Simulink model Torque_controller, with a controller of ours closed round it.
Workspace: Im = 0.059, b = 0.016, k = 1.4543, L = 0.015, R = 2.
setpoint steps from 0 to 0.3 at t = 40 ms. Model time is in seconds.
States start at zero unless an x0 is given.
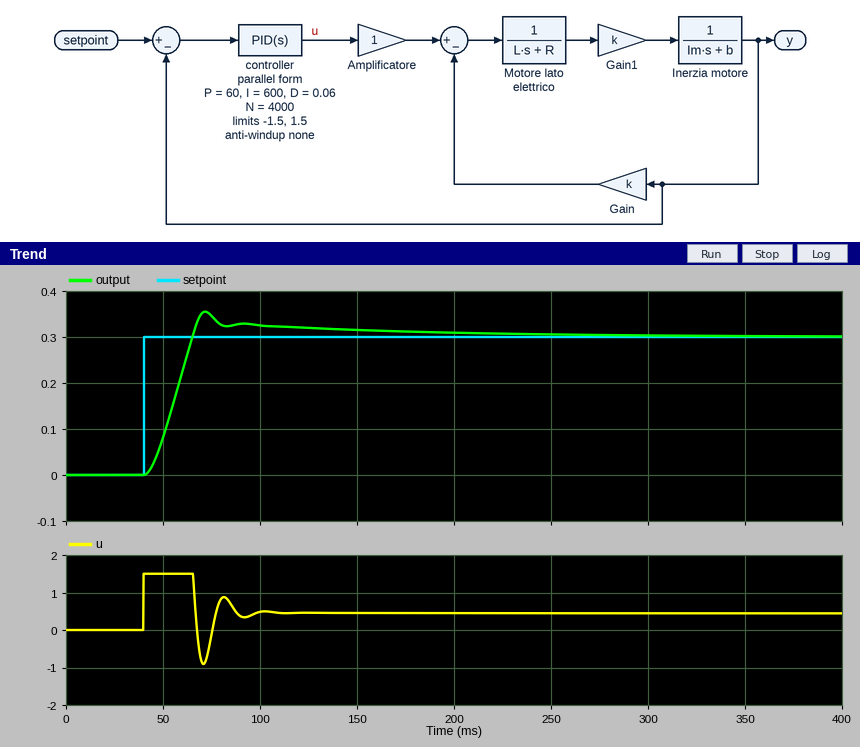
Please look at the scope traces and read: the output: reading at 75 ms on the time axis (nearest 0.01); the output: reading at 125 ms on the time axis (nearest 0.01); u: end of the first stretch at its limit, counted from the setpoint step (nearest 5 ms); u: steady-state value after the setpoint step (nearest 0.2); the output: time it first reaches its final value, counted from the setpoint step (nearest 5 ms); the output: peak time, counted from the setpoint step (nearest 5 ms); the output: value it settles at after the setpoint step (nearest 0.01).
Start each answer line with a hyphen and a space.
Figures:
- 0.35
- 0.32
- 25 ms
- 0.4
- 25 ms
- 30 ms
- 0.30
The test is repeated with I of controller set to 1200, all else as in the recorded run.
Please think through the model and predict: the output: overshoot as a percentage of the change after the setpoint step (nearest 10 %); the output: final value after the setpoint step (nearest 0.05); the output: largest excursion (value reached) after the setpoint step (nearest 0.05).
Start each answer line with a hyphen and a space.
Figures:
- 30 %
- 0.30
- 0.40
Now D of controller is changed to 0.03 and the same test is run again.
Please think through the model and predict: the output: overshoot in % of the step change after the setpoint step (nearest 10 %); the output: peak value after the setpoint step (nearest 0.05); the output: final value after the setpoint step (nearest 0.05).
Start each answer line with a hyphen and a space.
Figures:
- 20 %
- 0.35
- 0.30
